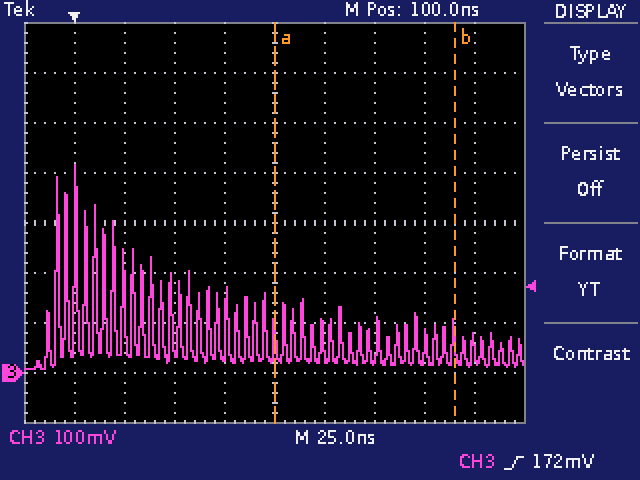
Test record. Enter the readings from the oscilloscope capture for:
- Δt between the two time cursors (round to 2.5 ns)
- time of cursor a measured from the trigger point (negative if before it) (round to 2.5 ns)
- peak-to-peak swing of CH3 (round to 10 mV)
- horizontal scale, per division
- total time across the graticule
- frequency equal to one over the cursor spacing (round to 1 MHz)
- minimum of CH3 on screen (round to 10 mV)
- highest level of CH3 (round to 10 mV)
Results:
90.0 ns
+100.0 ns
410 mV
25 ns
250 ns
11 MHz
10 mV
420 mV
